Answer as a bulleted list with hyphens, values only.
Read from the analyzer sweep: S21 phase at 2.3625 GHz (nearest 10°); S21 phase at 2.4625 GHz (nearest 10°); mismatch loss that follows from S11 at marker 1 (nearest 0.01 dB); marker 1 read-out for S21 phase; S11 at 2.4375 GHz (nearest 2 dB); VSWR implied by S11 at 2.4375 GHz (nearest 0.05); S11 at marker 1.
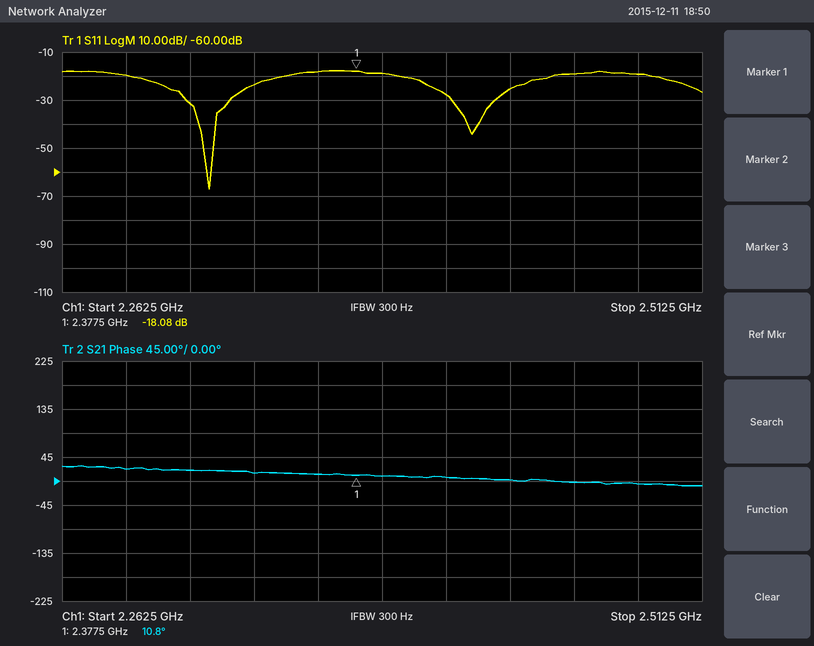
- 10°
- 0°
- 0.07 dB
- 10.8°
- -26 dB
- 1.10
- -18.08 dB
